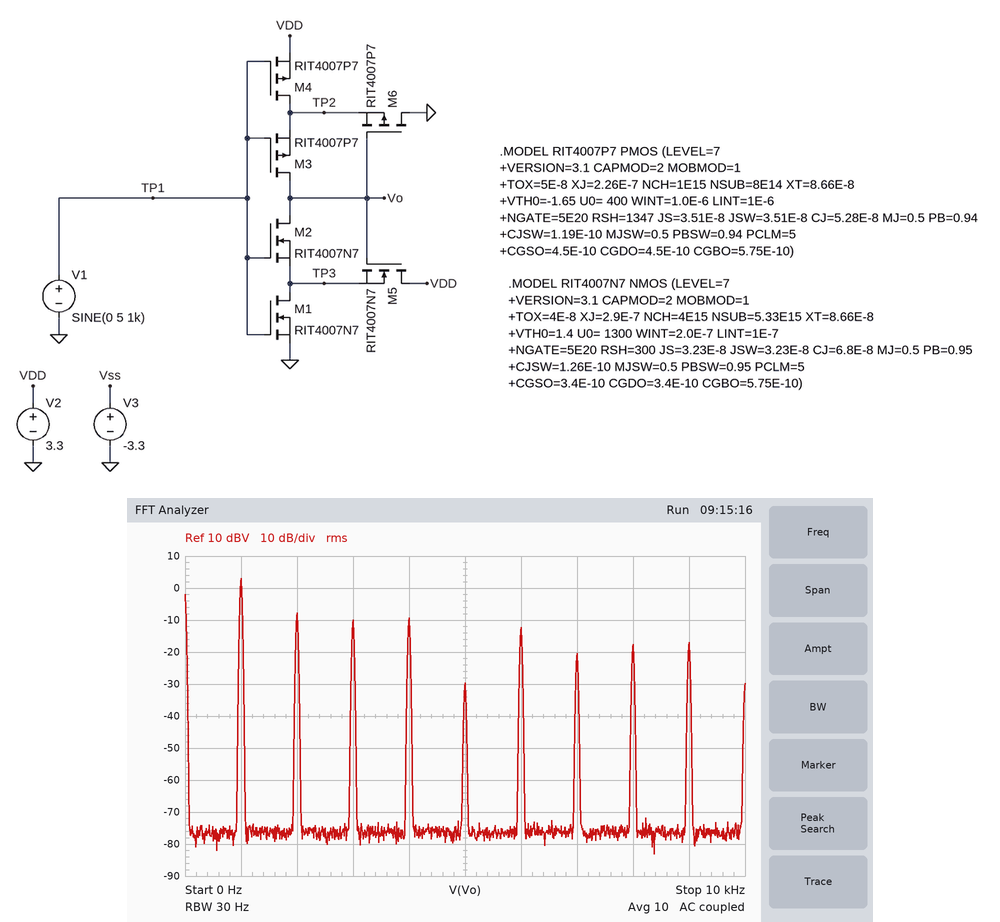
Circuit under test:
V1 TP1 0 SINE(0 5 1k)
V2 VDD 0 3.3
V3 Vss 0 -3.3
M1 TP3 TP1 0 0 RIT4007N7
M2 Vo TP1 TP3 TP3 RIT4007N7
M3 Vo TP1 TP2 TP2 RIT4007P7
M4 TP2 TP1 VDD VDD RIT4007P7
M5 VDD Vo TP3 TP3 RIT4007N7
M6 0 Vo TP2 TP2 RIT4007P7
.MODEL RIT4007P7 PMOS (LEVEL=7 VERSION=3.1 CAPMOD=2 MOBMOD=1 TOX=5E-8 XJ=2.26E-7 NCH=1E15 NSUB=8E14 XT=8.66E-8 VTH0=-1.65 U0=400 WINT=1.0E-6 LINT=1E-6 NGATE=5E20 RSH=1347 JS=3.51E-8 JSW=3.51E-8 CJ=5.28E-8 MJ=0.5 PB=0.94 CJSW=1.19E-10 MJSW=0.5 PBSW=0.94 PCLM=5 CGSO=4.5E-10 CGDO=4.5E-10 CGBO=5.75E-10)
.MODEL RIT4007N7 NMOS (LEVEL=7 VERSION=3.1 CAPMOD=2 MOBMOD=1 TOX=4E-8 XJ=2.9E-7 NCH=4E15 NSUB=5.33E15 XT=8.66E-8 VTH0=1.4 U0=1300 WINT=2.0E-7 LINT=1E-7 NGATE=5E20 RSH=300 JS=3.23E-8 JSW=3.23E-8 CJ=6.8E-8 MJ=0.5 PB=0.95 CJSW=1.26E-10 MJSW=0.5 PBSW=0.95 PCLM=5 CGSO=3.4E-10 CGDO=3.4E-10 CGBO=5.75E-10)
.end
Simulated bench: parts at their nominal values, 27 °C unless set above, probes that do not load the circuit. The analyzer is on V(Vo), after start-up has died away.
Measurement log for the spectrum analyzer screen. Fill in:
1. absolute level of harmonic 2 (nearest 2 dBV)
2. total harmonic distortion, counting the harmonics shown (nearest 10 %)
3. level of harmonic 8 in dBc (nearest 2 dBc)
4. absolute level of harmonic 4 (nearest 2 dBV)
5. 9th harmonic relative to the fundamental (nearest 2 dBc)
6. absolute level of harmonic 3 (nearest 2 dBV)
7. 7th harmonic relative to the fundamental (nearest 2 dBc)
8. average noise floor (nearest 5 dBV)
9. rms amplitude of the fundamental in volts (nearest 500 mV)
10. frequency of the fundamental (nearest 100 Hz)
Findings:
-8 dBV
50 %
-20 dBc
-10 dBV
-20 dBc
-10 dBV
-24 dBc
-75 dBV
1.5 V
1.0 kHz
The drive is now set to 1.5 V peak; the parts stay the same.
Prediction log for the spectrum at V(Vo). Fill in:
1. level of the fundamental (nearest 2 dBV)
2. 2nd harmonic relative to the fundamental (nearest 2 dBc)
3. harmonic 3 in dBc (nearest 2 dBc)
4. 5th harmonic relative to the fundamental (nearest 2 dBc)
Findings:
-32 dBV
0 dBc
0 dBc
-2 dBc
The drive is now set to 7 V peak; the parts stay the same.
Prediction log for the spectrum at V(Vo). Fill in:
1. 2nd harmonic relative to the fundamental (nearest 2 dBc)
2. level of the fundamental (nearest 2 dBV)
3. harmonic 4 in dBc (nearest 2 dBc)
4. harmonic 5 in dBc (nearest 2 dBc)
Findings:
-14 dBc
4 dBV
-14 dBc
-20 dBc
